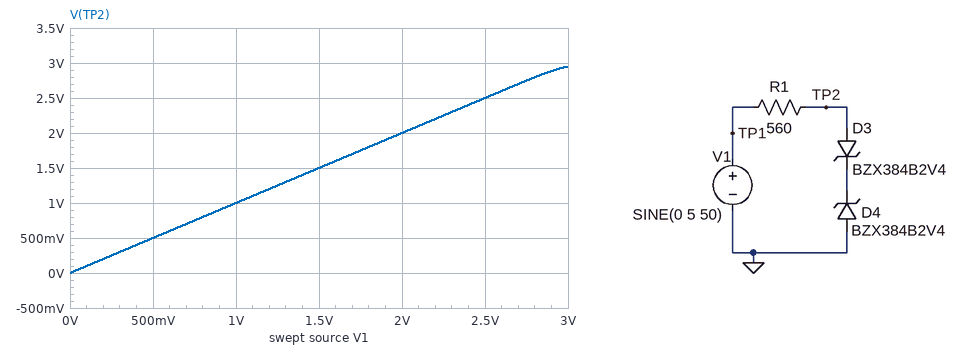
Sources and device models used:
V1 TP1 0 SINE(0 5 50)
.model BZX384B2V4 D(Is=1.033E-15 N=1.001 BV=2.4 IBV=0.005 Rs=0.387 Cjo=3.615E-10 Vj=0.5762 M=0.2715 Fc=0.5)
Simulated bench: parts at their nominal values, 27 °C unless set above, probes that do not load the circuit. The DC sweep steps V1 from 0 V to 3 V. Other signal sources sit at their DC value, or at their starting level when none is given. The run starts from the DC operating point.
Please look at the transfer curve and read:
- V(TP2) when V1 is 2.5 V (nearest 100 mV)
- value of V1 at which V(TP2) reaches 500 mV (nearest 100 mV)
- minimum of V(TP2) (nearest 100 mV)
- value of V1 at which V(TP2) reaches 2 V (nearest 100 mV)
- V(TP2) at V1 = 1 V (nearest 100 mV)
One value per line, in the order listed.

2.5 V
500 mV
0 V
2.0 V
1.0 V
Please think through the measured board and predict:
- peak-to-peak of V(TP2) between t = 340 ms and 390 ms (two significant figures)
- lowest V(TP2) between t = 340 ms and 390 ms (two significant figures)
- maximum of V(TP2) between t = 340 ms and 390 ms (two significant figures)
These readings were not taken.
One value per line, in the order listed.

6.3 V
-3.1 V
3.1 V
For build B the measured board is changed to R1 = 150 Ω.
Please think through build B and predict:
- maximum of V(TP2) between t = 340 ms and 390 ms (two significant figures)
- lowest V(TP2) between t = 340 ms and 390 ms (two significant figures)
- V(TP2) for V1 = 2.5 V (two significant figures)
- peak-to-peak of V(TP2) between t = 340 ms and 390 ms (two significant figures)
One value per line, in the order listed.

3.2 V
-3.2 V
2.5 V
6.4 V
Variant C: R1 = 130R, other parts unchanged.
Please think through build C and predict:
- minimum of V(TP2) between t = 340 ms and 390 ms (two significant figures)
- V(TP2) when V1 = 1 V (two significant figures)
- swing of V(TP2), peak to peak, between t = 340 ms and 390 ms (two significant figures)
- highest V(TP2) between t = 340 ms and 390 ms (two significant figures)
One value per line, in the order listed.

-3.2 V
1.0 V
6.4 V
3.2 V
